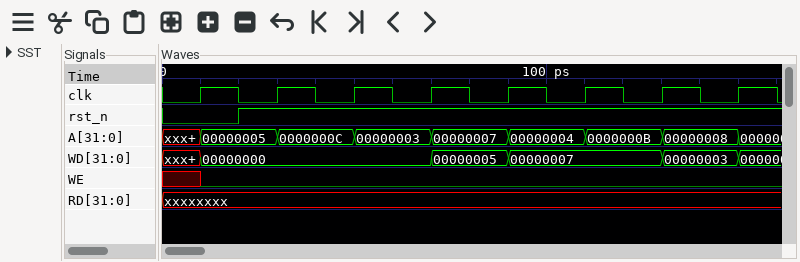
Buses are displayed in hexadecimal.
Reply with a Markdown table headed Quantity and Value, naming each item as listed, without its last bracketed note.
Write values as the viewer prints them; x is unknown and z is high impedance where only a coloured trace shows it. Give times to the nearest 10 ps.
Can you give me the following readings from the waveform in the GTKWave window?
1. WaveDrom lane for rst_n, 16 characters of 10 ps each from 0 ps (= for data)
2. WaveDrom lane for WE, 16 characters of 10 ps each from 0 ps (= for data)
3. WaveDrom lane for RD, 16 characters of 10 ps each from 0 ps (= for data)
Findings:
| Quantity | Value |
|---|---|
| WaveDrom lane for rst_n, 16 characters of 10 ps each from 0 ps | {name: 'rst_n', wave: '0.1.............'} |
| WaveDrom lane for WE, 16 characters of 10 ps each from 0 ps | {name: 'WE', wave: 'x0..............'} |
| WaveDrom lane for RD, 16 characters of 10 ps each from 0 ps | {name: 'RD', wave: 'x...............'} |
